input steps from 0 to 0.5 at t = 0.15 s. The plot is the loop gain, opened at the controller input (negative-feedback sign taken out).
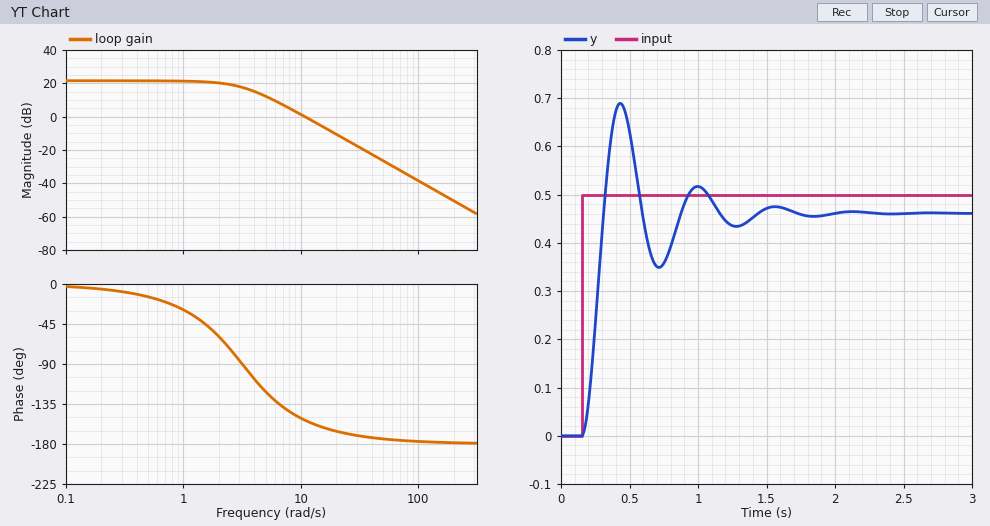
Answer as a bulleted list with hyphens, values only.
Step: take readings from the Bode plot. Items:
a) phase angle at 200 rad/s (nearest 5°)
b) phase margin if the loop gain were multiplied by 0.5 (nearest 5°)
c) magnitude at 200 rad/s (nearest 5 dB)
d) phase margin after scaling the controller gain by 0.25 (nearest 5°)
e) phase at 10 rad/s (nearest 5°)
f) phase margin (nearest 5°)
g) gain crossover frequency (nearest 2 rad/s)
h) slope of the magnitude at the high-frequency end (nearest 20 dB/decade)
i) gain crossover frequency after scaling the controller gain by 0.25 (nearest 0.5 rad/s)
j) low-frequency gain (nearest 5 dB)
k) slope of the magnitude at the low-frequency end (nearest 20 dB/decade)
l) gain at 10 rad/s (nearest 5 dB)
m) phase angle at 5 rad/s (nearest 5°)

- -180°
- 40°
- -50 dB
- 60°
- -150°
- 25°
- 10 rad/s
- -40 dB/decade
- 5.0 rad/s
- 20 dB
- 0 dB/decade
- 0 dB
- -120°
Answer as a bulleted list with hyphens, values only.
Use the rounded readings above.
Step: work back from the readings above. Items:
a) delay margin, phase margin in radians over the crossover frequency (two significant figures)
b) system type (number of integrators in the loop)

- 0.044 s
- 0
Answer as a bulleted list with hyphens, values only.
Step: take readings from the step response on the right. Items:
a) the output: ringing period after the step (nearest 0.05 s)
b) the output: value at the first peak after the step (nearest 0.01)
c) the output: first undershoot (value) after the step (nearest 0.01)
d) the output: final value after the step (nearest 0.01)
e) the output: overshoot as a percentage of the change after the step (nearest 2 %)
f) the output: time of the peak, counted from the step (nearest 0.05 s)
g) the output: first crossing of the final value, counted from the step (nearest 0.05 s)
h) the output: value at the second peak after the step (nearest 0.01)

- 0.55 s
- 0.69
- 0.35
- 0.46
- 50 %
- 0.30 s
- 0.15 s
- 0.52
